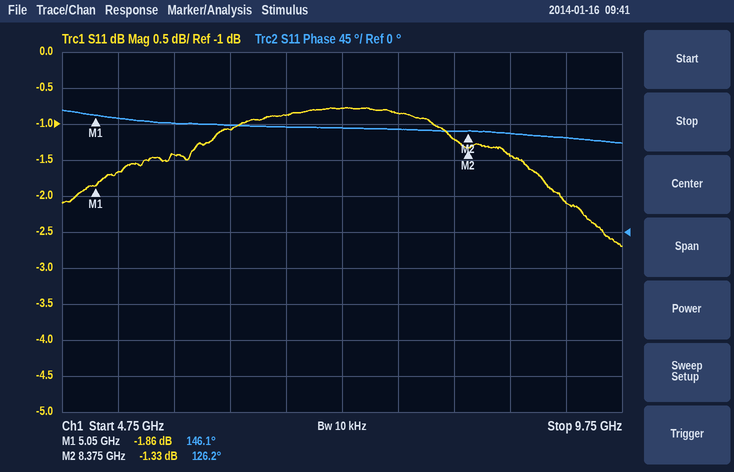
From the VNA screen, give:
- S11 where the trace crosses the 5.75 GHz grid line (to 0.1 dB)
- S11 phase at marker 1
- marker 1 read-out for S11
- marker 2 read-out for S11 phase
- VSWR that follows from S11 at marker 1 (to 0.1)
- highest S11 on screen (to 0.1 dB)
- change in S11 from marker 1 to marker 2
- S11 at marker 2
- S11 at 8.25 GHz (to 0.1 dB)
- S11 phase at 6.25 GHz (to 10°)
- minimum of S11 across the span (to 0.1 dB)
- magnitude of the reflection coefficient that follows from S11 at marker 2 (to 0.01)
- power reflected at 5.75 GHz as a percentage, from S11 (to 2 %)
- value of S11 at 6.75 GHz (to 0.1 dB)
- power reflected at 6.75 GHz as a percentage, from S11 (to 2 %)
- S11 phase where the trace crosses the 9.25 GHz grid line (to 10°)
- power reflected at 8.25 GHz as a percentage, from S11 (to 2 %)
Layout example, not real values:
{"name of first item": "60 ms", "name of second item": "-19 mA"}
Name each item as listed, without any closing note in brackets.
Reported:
{"S11 where the trace crosses the 5.75 GHz grid line": "-1.4 dB", "S11 phase at marker 1": "146.1°", "marker 1 read-out for S11": "-1.86 dB", "marker 2 read-out for S11 phase": "126.2°", "VSWR that follows from S11 at marker 1": "9.4", "highest S11 on screen": "-0.8 dB", "change in S11 from marker 1 to marker 2": "0.53 dB", "S11 at marker 2": "-1.33 dB", "S11 at 8.25 GHz": "-1.2 dB", "S11 phase at 6.25 GHz": "130°", "minimum of S11 across the span": "-2.7 dB", "magnitude of the reflection coefficient that follows from S11 at marker 2": "0.86", "power reflected at 5.75 GHz as a percentage, from S11": "72 %", "value of S11 at 6.75 GHz": "-0.9 dB", "power reflected at 6.75 GHz as a percentage, from S11": "82 %", "S11 phase where the trace crosses the 9.25 GHz grid line": "120°", "power reflected at 8.25 GHz as a percentage, from S11": "76 %"}
